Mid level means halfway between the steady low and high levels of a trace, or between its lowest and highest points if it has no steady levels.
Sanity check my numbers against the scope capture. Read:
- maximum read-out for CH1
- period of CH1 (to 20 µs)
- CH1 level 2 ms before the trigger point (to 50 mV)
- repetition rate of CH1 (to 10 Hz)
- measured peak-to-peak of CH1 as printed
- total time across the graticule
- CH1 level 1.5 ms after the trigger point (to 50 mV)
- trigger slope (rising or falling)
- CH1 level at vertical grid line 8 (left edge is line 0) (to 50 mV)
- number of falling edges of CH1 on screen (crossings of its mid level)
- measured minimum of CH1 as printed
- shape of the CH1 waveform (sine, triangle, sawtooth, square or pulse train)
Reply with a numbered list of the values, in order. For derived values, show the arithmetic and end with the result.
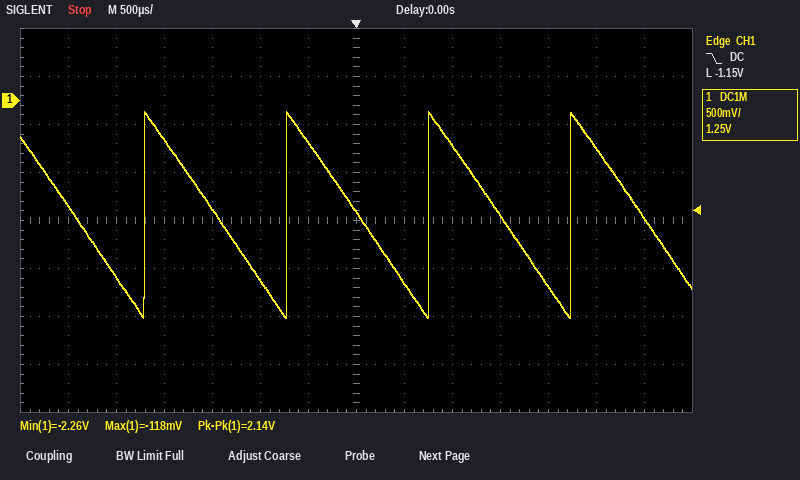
1. -118 mV
2. 1.48 ms
3. -400 mV
4. 1 / 1.48 ms ≈ 676 Hz, so 680 Hz to the nearest 10 Hz
5. 2.14 V
6. 7 ms
7. -1.20 V
8. falling
9. -1.90 V
10. 5
11. -2.26 V
12. sawtooth
